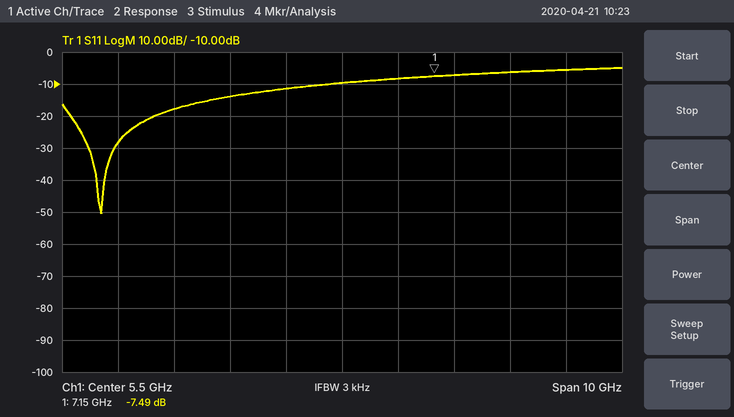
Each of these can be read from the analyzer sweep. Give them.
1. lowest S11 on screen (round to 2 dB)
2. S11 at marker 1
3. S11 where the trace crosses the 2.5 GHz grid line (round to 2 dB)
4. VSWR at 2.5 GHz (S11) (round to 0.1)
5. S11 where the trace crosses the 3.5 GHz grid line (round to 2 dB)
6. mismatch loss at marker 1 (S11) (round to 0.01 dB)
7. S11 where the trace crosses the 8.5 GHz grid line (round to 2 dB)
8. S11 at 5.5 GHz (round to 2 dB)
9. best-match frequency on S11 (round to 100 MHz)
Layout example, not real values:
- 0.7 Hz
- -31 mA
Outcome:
- -50 dB
- -7.49 dB
- -18 dB
- 1.3
- -14 dB
- 0.85 dB
- -6 dB
- -10 dB
- 1.2 GHz
